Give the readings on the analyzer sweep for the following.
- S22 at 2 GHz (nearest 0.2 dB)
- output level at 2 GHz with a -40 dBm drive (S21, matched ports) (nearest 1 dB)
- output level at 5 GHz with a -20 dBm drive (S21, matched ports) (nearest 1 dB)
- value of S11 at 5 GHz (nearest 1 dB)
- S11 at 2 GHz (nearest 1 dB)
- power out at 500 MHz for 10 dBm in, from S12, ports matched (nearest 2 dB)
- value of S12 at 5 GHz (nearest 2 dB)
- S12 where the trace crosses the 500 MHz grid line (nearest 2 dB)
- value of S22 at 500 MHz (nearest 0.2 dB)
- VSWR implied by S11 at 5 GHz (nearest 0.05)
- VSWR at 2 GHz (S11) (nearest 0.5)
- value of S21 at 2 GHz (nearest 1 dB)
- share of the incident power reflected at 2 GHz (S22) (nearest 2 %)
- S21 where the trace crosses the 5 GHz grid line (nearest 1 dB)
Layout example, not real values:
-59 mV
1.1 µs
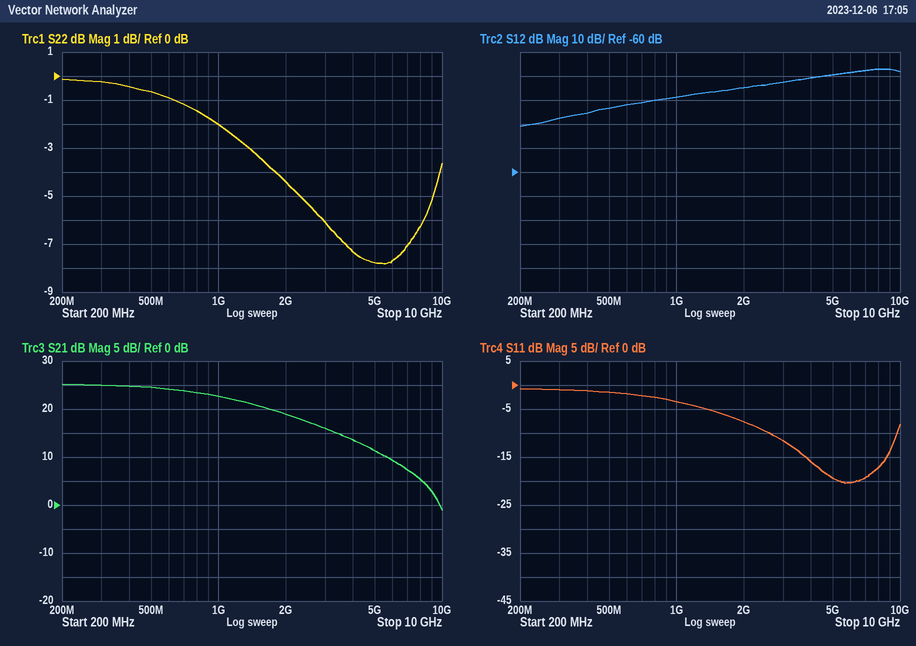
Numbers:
-4.4 dB
-21 dBm
-9 dBm
-19 dB
-8 dB
-24 dBm
-20 dB
-34 dB
-0.6 dB
1.25
2.5
19 dB
36 %
11 dB
